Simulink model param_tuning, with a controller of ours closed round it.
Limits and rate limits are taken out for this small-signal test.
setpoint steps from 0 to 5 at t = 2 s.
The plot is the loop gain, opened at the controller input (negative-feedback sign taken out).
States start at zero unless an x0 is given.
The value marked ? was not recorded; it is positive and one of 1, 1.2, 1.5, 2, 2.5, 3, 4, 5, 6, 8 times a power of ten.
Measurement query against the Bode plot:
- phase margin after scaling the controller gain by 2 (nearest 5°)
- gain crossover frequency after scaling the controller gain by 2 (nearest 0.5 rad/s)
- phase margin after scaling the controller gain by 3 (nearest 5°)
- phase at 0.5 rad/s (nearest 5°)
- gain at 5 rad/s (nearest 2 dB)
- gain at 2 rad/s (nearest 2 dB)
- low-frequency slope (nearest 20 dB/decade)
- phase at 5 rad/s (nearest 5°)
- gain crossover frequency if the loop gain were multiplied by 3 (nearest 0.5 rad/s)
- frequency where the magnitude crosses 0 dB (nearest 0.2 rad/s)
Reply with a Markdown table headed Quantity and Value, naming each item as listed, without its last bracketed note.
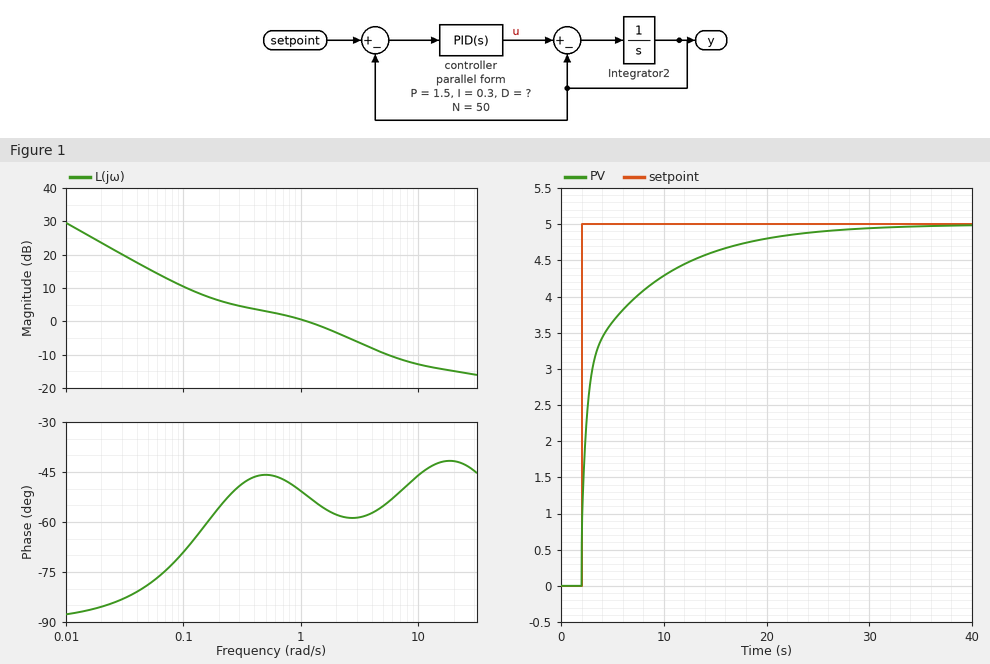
| Quantity | Value |
|---|---|
| phase margin after scaling the controller gain by 2 | 120° |
| gain crossover frequency after scaling the controller gain by 2 | 3.0 rad/s |
| phase margin after scaling the controller gain by 3 | 125° |
| phase at 0.5 rad/s | -45° |
| gain at 5 rad/s | -10 dB |
| gain at 2 rad/s | -4 dB |
| low-frequency slope | -20 dB/decade |
| phase at 5 rad/s | -55° |
| gain crossover frequency if the loop gain were multiplied by 3 | 5.0 rad/s |
| frequency where the magnitude crosses 0 dB | 1.2 rad/s |
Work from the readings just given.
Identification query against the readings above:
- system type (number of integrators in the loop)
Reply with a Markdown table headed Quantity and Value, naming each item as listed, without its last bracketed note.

| Quantity | Value |
|---|---|
| system type | 1 |
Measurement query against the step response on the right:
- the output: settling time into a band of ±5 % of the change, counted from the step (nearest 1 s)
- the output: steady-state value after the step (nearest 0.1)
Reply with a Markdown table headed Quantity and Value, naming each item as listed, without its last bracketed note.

| Quantity | Value |
|---|---|
| the output: settling time into a band of ±5 % of the change, counted from the step | 16 s |
| the output: steady-state value after the step | 5.0 |
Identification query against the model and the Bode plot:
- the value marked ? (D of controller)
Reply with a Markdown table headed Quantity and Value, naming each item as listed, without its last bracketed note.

| Quantity | Value |
|---|---|
| the value marked ? | 0.15 |
